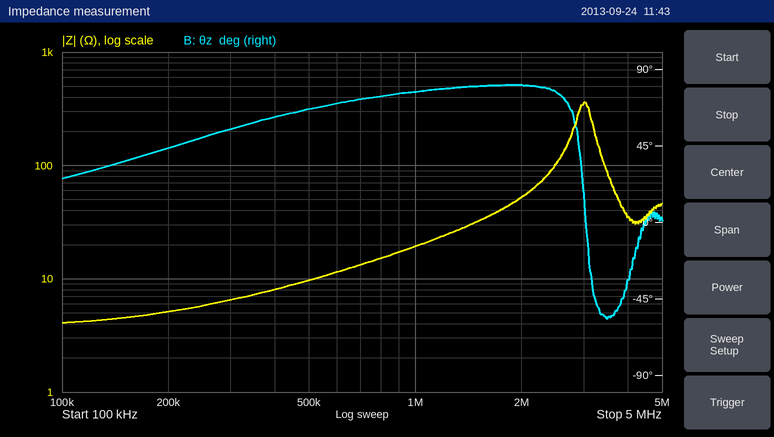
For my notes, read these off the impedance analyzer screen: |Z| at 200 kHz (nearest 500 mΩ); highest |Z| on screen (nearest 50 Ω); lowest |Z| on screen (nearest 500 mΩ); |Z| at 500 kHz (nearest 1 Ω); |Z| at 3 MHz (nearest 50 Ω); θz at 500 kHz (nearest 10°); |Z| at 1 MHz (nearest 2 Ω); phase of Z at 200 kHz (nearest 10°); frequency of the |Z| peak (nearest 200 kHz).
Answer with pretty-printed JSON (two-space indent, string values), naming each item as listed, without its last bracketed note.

{
  "|Z| at 200 kHz": "5.0 Ω",
  "highest |Z| on screen": "350 Ω",
  "lowest |Z| on screen": "4.0 Ω",
  "|Z| at 500 kHz": "10 Ω",
  "|Z| at 3 MHz": "350 Ω",
  "θz at 500 kHz": "70°",
  "|Z| at 1 MHz": "20 Ω",
  "phase of Z at 200 kHz": "40°",
  "frequency of the |Z| peak": "3.0 MHz"
}
